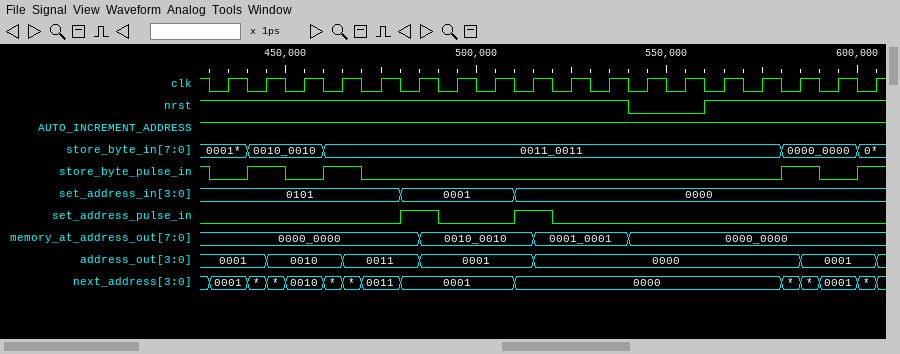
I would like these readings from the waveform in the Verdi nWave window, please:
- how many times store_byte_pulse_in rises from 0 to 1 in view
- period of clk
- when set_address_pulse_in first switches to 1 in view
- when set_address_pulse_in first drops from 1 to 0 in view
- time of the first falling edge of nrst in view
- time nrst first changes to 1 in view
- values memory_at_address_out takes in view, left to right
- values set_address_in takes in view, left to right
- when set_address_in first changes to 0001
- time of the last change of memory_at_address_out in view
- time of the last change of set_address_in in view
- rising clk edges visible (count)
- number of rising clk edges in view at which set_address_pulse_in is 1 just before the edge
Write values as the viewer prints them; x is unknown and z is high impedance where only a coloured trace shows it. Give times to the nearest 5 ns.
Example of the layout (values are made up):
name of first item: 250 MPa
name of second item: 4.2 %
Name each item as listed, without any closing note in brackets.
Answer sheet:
how many times store_byte_pulse_in rises from 0 to 1 in view: 4
period of clk: 10 ns
when set_address_pulse_in first switches to 1 in view: 480 ns
when set_address_pulse_in first drops from 1 to 0 in view: 490 ns
time of the first falling edge of nrst in view: 540 ns
time nrst first changes to 1 in view: 560 ns
values memory_at_address_out takes in view, left to right: 0000_0000, 0010_0010, 0001_0001, 0000_0000
values set_address_in takes in view, left to right: 0101, 0001, 0000
when set_address_in first changes to 0001: 480 ns
time of the last change of memory_at_address_out in view: 540 ns
time of the last change of set_address_in in view: 510 ns
rising clk edges visible: 18
number of rising clk edges in view at which set_address_pulse_in is 1 just before the edge: 2
